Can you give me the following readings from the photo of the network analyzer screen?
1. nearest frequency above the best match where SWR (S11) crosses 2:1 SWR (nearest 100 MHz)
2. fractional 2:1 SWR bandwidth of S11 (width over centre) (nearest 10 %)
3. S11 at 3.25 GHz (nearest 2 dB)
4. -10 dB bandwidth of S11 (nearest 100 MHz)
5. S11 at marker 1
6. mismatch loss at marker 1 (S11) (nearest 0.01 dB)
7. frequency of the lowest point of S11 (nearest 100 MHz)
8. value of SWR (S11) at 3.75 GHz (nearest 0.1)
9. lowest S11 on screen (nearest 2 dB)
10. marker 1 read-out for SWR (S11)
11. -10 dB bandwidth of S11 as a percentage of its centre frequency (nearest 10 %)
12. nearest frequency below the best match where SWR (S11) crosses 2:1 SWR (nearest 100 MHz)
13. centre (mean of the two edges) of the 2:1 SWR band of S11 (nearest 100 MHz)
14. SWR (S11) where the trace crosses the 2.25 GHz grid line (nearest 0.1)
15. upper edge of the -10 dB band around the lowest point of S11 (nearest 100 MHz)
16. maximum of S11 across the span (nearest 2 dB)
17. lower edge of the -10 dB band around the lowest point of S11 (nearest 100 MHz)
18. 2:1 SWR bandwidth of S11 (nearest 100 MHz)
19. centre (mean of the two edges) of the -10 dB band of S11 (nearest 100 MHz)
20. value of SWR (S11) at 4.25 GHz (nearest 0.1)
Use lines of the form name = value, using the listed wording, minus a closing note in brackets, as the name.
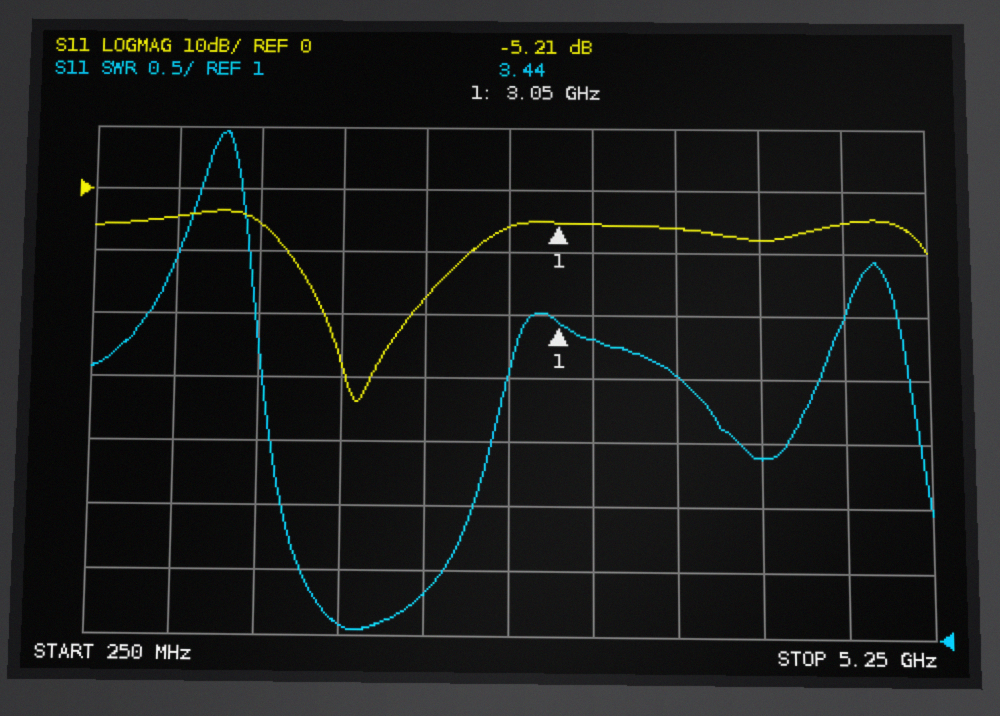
nearest frequency above the best match where SWR (S11) crosses 2:1 SWR = 2.5 GHz
fractional 2:1 SWR bandwidth of S11 (width over centre) = 60 %
S11 at 3.25 GHz = -6 dB
-10 dB bandwidth of S11 = 1.1 GHz
S11 at marker 1 = -5.21 dB
mismatch loss at marker 1 (S11) = 1.56 dB
frequency of the lowest point of S11 = 1.8 GHz
value of SWR (S11) at 3.75 GHz = 3.0
lowest S11 on screen = -34 dB
marker 1 read-out for SWR = 3.44
-10 dB bandwidth of S11 as a percentage of its centre frequency = 60 %
nearest frequency below the best match where SWR (S11) crosses 2:1 SWR = 1.4 GHz
centre (mean of the two edges) of the 2:1 SWR band of S11 = 2.0 GHz
SWR (S11) where the trace crosses the 2.25 GHz grid line = 1.3
upper edge of the -10 dB band around the lowest point of S11 = 2.5 GHz
maximum of S11 across the span = -4 dB
lower edge of the -10 dB band around the lowest point of S11 = 1.4 GHz
2:1 SWR bandwidth of S11 = 1.1 GHz
centre (mean of the two edges) of the -10 dB band of S11 = 2.0 GHz
value of SWR (S11) at 4.25 GHz = 2.4
